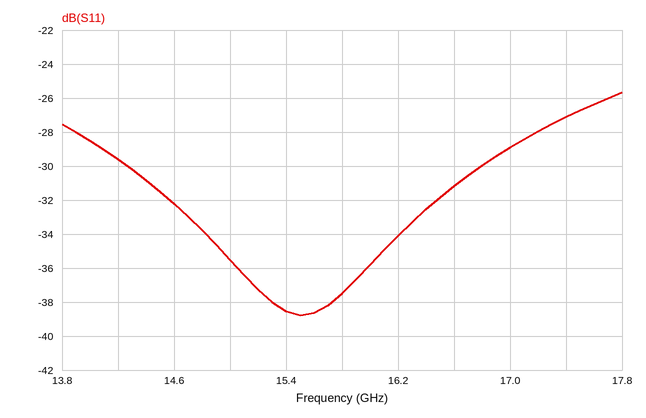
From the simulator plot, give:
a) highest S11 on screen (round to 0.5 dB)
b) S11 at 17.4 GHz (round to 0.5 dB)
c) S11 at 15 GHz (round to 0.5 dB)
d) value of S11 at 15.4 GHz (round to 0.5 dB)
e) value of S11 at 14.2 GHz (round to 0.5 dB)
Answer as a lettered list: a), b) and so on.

a) -25.5 dB
b) -27.0 dB
c) -35.5 dB
d) -38.5 dB
e) -29.5 dB
